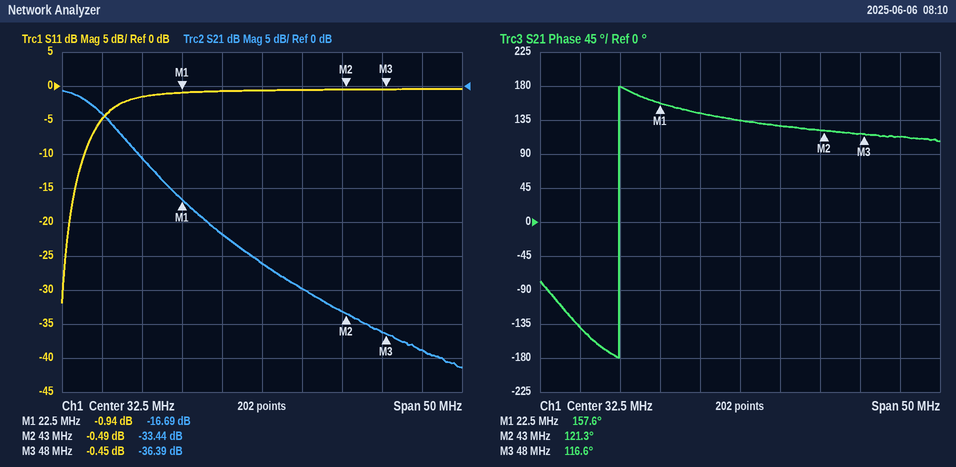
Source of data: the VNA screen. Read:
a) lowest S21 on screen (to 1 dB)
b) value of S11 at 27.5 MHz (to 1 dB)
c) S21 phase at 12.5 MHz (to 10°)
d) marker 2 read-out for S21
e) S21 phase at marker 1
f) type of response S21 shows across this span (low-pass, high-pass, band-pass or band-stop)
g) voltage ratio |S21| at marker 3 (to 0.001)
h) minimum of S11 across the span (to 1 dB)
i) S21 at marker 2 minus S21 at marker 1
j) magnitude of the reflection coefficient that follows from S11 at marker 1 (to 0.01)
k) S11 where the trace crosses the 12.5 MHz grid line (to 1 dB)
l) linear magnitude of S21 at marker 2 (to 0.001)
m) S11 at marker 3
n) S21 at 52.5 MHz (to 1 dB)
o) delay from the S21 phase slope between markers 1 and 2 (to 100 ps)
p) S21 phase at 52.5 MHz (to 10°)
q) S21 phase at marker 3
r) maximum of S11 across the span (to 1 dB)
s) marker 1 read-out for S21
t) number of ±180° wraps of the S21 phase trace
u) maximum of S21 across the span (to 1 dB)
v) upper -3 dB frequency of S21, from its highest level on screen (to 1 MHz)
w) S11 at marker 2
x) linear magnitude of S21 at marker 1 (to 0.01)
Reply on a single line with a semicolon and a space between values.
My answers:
-41 dB; -1 dB; -140°; -33.44 dB; 157.6°; low-pass; 0.015; -32 dB; -16.75 dB; 0.90; -5 dB; 0.021; -0.45 dB; -39 dB; 4.9 ns; 110°; 116.6°; 0 dB; -16.69 dB; 1; -1 dB; 12 MHz; -0.49 dB; 0.15
